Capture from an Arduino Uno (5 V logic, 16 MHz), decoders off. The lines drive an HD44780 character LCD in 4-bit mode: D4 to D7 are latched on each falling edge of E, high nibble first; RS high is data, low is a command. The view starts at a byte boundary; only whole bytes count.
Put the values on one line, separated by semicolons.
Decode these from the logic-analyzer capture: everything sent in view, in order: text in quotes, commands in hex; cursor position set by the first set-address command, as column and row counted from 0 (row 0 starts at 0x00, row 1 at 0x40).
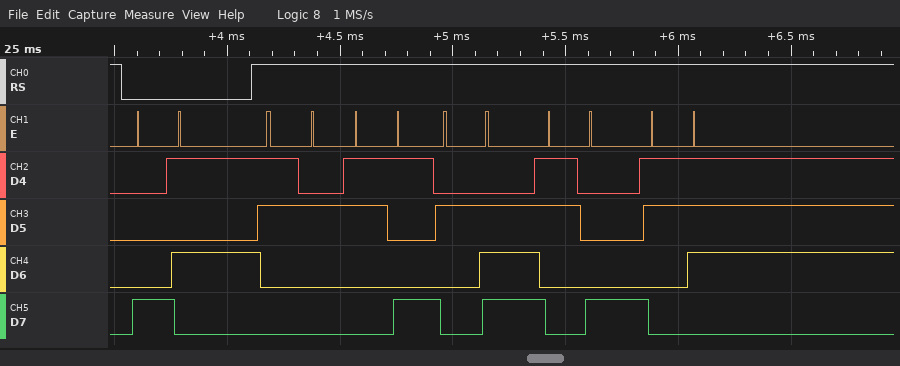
0x85 "29.87"; column 5, row 0
